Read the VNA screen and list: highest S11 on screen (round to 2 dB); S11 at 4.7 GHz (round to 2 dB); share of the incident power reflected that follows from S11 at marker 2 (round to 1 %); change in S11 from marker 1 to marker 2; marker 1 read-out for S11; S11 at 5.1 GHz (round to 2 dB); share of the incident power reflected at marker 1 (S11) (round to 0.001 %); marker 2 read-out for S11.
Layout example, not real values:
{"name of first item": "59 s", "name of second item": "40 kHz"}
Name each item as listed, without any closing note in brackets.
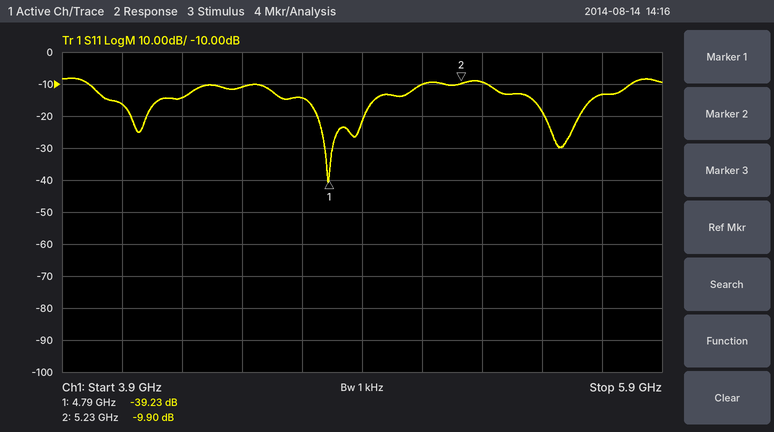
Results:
{"highest S11 on screen": "-8 dB", "S11 at 4.7 GHz": "-14 dB", "share of the incident power reflected that follows from S11 at marker 2": "10 %", "change in S11 from marker 1 to marker 2": "29.33 dB", "marker 1 read-out for S11": "-39.23 dB", "S11 at 5.1 GHz": "-10 dB", "share of the incident power reflected at marker 1 (S11)": "0.012 %", "marker 2 read-out for S11": "-9.90 dB"}
